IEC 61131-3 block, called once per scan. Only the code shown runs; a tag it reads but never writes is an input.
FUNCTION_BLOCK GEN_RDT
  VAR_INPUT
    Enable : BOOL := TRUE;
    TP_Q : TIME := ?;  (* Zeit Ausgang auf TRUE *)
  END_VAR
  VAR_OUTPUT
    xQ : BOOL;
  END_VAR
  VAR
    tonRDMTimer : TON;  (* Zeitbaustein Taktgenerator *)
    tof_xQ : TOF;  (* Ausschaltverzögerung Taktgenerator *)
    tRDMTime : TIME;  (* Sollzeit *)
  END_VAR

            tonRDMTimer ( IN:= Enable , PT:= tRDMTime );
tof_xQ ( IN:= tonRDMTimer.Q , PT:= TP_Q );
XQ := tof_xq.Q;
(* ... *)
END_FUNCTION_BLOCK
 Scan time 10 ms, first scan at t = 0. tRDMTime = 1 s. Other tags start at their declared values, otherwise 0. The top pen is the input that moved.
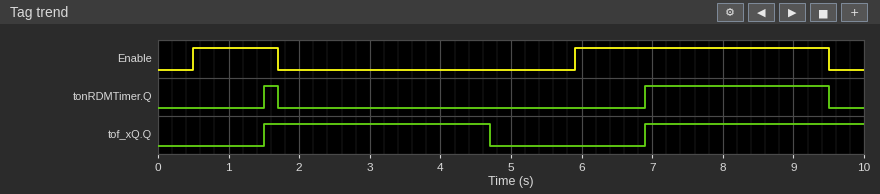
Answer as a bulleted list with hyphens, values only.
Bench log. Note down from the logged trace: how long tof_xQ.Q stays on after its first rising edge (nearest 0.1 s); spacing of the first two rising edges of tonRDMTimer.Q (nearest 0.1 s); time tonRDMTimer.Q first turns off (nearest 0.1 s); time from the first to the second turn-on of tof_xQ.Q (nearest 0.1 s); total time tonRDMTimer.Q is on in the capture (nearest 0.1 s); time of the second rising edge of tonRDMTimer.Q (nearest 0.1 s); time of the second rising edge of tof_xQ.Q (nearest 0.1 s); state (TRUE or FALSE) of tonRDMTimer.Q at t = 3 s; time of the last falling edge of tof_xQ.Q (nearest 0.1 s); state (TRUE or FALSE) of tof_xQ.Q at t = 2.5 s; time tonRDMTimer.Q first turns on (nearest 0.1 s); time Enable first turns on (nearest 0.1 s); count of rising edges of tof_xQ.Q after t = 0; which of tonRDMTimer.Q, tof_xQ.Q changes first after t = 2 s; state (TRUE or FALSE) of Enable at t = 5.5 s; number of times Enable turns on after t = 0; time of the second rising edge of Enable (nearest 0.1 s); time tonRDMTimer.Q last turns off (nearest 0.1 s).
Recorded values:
- 3.2 s
- 5.4 s
- 1.7 s
- 5.4 s
- 2.8 s
- 6.9 s
- 6.9 s
- FALSE
- 4.7 s
- TRUE
- 1.5 s
- 0.5 s
- 2
- tof_xQ.Q
- FALSE
- 2
- 5.9 s
- 9.5 s
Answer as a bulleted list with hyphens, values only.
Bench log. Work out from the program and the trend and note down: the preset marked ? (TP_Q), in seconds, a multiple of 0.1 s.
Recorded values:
- 3.0 s
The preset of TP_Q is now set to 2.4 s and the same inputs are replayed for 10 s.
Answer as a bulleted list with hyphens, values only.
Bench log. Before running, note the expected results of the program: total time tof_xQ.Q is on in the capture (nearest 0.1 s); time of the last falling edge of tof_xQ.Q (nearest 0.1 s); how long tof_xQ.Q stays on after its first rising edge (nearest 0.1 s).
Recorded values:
- 5.7 s
- 4.1 s
- 2.6 s
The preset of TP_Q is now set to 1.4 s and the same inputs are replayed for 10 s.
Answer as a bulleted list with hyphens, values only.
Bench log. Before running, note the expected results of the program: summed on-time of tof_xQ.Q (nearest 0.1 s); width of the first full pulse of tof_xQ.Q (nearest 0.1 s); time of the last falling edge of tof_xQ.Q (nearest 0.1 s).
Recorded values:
- 4.7 s
- 1.6 s
- 3.1 s
